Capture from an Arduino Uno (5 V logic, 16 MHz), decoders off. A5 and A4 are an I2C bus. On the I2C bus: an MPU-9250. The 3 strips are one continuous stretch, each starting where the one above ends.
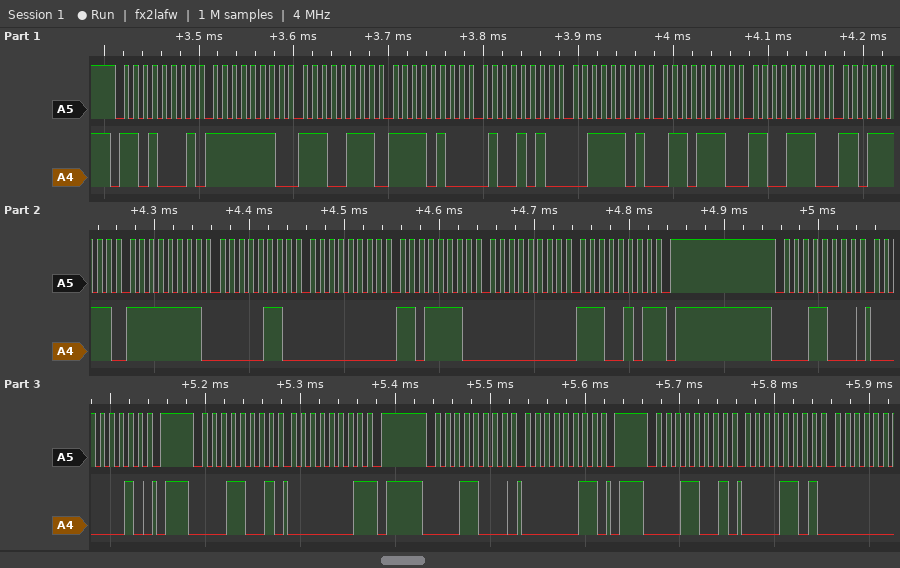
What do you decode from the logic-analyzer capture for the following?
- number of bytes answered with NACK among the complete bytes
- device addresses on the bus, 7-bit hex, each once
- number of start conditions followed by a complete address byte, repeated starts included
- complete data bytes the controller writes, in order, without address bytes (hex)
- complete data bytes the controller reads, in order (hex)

2
0x68 0x0C
5
02 03
FE E7 F4 4A 3D 6E CE DF FF 06 00 DE 00 E5 01 0D
